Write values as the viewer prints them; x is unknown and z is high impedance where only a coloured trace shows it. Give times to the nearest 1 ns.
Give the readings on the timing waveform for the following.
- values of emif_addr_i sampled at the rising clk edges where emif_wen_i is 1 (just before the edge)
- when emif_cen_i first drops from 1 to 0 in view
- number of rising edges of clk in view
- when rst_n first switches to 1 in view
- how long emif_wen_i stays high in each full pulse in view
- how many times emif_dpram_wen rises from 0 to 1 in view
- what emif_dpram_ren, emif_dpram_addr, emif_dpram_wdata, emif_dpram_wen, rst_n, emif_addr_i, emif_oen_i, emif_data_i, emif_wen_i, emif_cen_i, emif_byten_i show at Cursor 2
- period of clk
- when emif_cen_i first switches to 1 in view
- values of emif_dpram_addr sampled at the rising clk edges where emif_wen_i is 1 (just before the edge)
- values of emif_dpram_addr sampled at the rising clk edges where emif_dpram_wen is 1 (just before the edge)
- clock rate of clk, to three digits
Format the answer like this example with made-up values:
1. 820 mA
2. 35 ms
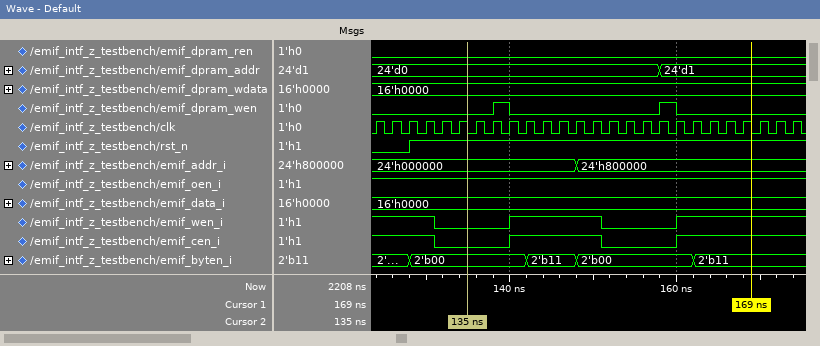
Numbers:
1. 24'h000000, 24'h000000, 24'h000000, 24'h000000, 24'h000000, 24'h000000, 24'h000000, 24'h000000, 24'h800000, 24'h800000, 24'h800000, 24'h800000, 24'h800000, 24'h800000, 24'h800000, 24'h800000
2. 131 ns
3. 26
4. 128 ns
5. 11 ns
6. 2
7. emif_dpram_ren=0, emif_dpram_addr=24'd0, emif_dpram_wdata=16'h0000, emif_dpram_wen=0, rst_n=1, emif_addr_i=24'h000000, emif_oen_i=1, emif_data_i=16'h0000, emif_wen_i=0, emif_cen_i=0, emif_byten_i=2'b00
8. 2 ns
9. 140 ns
10. 24'd0, 24'd0, 24'd0, 24'd0, 24'd0, 24'd0, 24'd0, 24'd0, 24'd0, 24'd1, 24'd1, 24'd1, 24'd1, 24'd1, 24'd1, 24'd1
11. 24'd0, 24'd1
12. 500 MHz
